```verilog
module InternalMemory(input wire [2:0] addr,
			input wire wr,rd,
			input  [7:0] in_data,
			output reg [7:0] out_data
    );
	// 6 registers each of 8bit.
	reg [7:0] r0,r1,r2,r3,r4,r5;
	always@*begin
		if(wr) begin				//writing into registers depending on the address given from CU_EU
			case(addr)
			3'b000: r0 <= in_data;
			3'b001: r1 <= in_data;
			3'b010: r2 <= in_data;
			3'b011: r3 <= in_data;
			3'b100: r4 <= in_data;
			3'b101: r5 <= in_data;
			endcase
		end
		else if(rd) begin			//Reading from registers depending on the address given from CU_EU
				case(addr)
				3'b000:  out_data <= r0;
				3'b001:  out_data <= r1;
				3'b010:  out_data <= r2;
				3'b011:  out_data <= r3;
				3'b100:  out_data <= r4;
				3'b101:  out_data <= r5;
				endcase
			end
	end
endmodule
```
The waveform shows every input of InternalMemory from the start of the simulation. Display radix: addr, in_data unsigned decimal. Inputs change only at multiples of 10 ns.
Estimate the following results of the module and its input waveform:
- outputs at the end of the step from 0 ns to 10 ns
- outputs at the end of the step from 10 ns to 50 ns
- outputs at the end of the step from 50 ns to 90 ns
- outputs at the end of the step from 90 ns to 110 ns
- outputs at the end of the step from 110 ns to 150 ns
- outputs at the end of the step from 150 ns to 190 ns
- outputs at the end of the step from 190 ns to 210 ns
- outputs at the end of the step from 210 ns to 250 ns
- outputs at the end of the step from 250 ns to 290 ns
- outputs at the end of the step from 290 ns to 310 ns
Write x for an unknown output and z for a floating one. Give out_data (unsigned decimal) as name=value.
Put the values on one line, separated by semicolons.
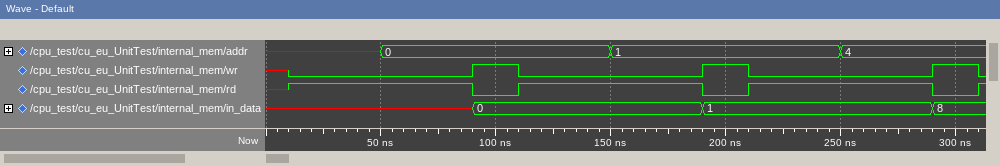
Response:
out_data=x; out_data=x; out_data=x; out_data=x; out_data=0; out_data=x; out_data=x; out_data=1; out_data=x; out_data=x
